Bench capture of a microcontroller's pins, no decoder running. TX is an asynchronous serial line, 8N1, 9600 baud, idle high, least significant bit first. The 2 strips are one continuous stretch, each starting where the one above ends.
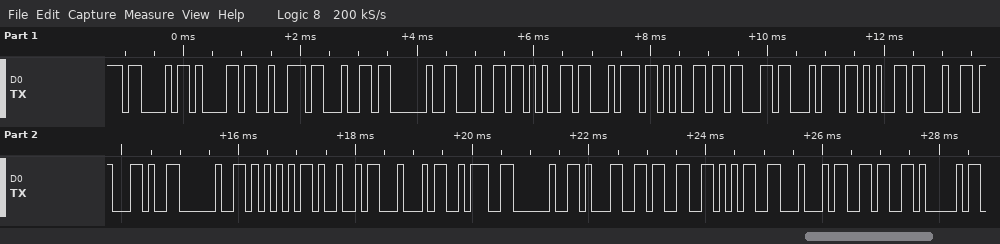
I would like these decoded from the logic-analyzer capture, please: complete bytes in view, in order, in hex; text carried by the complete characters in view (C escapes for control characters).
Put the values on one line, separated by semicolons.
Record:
43 61 72 64 20 64 65 74 65 63 74 65 64 2C 20 55 49 44 3A 20 31 33 35 44 36 41; "Card detected, UID: 135D6A"
